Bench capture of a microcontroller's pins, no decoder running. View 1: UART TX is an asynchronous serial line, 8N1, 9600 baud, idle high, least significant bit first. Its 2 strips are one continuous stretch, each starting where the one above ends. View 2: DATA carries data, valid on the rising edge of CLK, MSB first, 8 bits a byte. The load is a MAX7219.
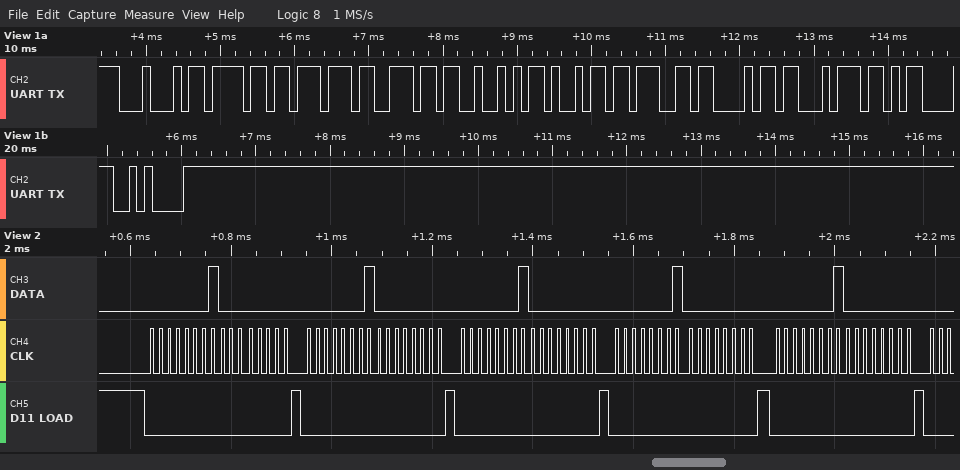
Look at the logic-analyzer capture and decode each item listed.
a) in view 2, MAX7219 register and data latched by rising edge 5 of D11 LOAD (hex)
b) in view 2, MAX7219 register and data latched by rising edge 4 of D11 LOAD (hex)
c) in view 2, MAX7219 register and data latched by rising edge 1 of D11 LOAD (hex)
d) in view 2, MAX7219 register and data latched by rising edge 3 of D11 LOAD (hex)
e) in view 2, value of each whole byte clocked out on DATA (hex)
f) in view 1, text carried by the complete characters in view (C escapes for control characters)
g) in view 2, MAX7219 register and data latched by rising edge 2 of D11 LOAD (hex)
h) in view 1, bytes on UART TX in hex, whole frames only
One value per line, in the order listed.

register 0x1, data 0x00
register 0x1, data 0x00
register 0x1, data 0x00
register 0x1, data 0x00
01 00 01 00 01 00 01 00 01 00
"DownRight\r\n"
register 0x1, data 0x00
0x44 0x6F 0x77 0x6E 0x52 0x69 0x67 0x68 0x74 0x0D 0x0A
